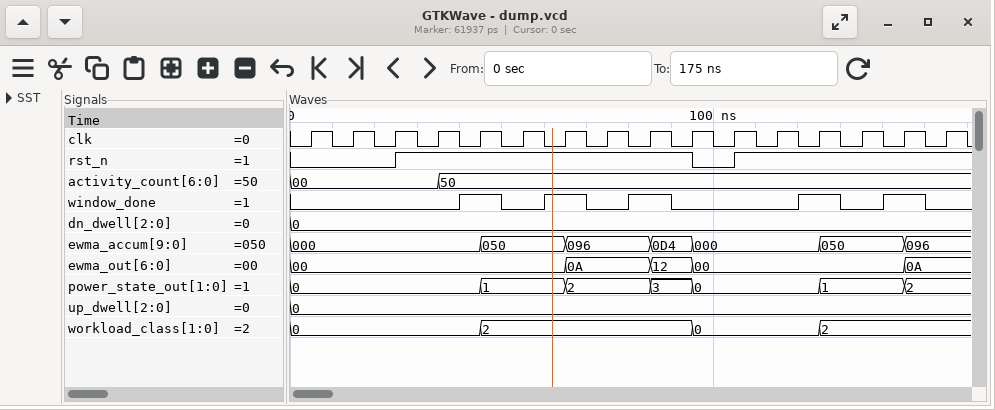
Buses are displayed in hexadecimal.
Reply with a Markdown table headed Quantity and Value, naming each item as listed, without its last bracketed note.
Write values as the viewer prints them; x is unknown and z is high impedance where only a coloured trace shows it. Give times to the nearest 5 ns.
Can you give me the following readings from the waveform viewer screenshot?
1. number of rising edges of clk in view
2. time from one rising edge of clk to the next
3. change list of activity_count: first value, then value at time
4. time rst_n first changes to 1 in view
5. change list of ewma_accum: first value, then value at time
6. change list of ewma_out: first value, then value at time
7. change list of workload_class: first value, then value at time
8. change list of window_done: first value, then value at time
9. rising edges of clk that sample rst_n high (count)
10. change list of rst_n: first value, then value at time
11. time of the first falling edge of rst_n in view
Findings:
| Quantity | Value |
|---|---|
| number of rising edges of clk in view | 16 |
| time from one rising edge of clk to the next | 10 ns |
| change list of activity_count: first value, then value at time | 00, 50 at 35 ns |
| time rst_n first changes to 1 in view | 25 ns |
| change list of ewma_accum: first value, then value at time | 000, 050 at 45 ns, 096 at 65 ns, 0D4 at 85 ns, 000 at 95 ns, 050 at 125 ns, 096 at 145 ns |
| change list of ewma_out: first value, then value at time | 00, 0A at 65 ns, 12 at 85 ns, 00 at 95 ns, 0A at 145 ns |
| change list of workload_class: first value, then value at time | 0, 2 at 45 ns, 0 at 95 ns, 2 at 125 ns |
| change list of window_done: first value, then value at time | 0, 1 at 40 ns, 0 at 50 ns, 1 at 60 ns, 0 at 70 ns, 1 at 80 ns, 0 at 90 ns, 1 at 120 ns, 0 at 130 ns, 1 at 140 ns, 0 at 150 ns |
| rising edges of clk that sample rst_n high | 12 |
| change list of rst_n: first value, then value at time | 0, 1 at 25 ns, 0 at 95 ns, 1 at 105 ns |
| time of the first falling edge of rst_n in view | 95 ns |
